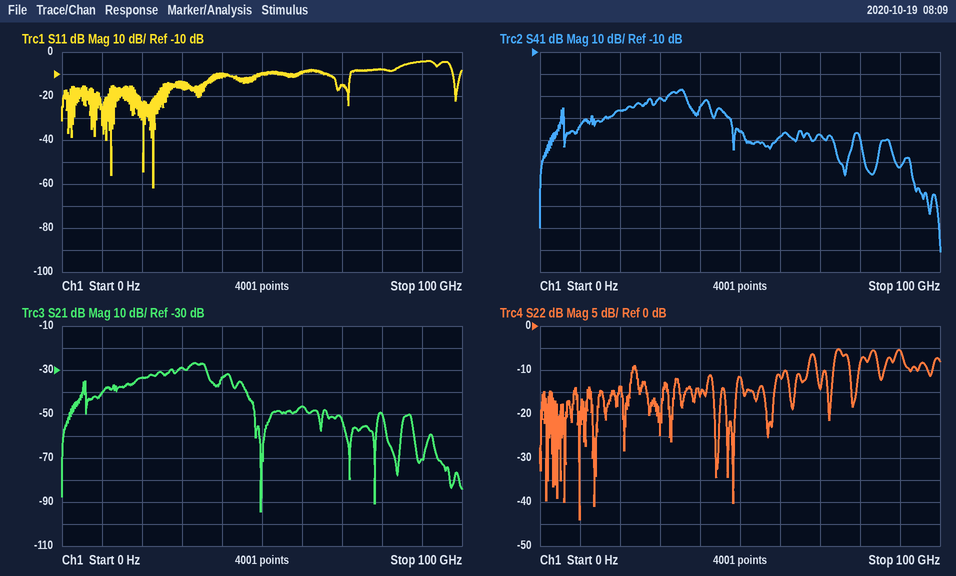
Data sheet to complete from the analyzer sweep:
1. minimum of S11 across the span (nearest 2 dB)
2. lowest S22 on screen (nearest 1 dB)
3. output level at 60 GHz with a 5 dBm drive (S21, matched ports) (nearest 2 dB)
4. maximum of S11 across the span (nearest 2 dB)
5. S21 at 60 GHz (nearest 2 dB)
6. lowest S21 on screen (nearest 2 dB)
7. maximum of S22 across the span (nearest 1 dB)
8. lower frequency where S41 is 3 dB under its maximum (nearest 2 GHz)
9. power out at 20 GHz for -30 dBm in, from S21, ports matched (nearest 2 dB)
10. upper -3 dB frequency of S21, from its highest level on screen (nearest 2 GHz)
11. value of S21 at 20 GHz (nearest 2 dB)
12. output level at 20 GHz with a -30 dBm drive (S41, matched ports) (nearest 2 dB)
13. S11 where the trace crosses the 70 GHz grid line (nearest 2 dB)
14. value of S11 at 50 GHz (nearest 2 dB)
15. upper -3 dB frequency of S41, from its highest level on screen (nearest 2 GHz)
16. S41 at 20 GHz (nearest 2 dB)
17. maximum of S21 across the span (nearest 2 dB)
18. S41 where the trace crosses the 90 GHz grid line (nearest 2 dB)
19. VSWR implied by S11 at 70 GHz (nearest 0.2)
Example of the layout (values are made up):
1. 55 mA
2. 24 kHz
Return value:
1. -62 dB
2. -44 dB
3. -42 dBm
4. -4 dB
5. -46 dB
6. -94 dB
7. -5 dB
8. 32 GHz
9. -64 dBm
10. 36 GHz
11. -34 dB
12. -66 dBm
13. -16 dB
14. -10 dB
15. 36 GHz
16. -36 dB
17. -26 dB
18. -62 dB
19. 1.4
